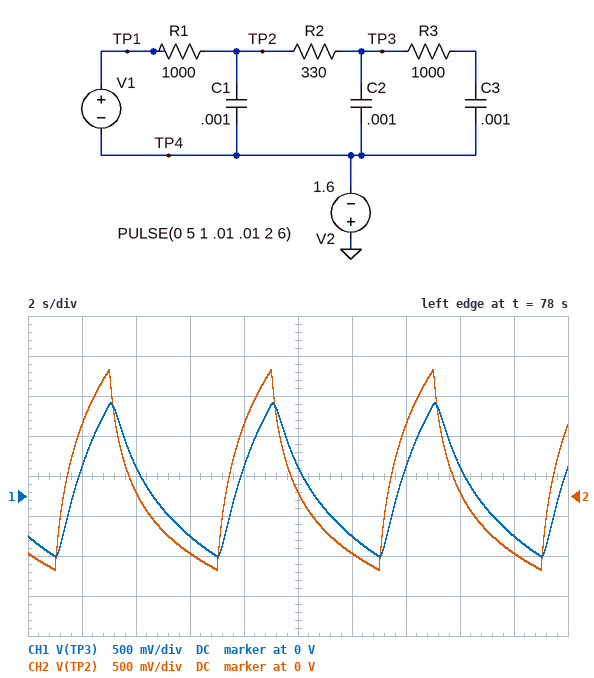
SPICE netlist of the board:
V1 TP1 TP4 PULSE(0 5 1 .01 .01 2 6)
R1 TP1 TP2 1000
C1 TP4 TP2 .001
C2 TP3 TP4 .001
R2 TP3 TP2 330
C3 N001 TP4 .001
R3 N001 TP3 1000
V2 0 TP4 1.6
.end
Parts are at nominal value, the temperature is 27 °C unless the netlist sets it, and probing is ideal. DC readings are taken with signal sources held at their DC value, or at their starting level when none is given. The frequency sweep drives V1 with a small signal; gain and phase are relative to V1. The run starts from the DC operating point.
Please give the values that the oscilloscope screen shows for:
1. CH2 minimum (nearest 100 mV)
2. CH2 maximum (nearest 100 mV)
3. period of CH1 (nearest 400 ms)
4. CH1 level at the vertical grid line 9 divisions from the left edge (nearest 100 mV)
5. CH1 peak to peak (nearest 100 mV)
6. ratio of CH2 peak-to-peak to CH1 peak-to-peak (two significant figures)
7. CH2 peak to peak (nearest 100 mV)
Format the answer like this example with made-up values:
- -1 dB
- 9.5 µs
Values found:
- -900 mV
- 1.6 V
- 6.0 s
- -500 mV
- 1.9 V
- 1.3
- 2.5 V
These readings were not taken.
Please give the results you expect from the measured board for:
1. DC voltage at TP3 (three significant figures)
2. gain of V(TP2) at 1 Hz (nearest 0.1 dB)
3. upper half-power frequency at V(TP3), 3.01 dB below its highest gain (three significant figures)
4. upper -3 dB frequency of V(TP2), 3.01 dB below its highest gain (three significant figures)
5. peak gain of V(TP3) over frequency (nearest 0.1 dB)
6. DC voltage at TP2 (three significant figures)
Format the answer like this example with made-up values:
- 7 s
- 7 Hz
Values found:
- -1.60 V
- -18.1 dB
- 42.3 mHz
- 45.9 mHz
- 0 dB
- -1.60 V
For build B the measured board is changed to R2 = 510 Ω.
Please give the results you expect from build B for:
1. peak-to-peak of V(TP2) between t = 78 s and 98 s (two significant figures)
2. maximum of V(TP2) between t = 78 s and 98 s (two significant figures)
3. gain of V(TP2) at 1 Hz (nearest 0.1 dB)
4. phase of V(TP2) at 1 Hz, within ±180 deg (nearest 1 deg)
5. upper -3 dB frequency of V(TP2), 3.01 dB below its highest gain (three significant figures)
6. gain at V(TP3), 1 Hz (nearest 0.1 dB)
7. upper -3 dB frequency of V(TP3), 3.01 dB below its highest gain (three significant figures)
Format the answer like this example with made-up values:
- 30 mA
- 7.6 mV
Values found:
- 2.6 V
- 1.7 V
- -17.3 dB
- -68 deg
- 44.9 mHz
- -28.4 dB
- 39.1 mHz
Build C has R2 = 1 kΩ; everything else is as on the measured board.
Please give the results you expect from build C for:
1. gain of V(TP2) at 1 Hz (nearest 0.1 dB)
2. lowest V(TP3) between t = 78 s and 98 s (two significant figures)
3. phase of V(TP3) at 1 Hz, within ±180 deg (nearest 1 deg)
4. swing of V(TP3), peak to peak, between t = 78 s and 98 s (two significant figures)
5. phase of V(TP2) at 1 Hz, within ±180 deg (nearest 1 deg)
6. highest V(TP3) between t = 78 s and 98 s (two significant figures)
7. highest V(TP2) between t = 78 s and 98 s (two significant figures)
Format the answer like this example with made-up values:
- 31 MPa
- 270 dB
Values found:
- -16.5 dB
- -550 mV
- -146 deg
- 1.4 V
- -73 deg
- 820 mV
- 1.9 V
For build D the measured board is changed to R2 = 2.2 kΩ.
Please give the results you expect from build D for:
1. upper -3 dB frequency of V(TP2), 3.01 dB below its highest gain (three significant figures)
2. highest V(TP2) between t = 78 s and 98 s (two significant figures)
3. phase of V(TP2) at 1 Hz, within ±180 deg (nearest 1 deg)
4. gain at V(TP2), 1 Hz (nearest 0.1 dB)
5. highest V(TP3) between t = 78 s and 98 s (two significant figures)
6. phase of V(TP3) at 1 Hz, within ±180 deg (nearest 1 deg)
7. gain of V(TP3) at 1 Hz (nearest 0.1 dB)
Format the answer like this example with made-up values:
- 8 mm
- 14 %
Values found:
- 57.9 mHz
- 2.2 V
- -77 deg
- -16.2 dB
- 530 mV
- -155 deg
- -39.5 dB
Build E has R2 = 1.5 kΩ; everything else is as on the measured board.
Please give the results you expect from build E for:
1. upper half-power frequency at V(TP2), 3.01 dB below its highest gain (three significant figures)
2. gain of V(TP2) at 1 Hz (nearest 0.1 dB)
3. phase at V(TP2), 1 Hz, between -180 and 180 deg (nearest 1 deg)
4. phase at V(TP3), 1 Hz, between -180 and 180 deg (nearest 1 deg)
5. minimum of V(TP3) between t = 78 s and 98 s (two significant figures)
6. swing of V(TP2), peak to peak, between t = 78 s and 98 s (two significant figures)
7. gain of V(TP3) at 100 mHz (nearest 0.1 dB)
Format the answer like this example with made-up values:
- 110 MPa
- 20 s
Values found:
- 47.0 mHz
- -16.3 dB
- -75 deg
- -151 deg
- -450 mV
- 3.1 V
- -11.3 dB
